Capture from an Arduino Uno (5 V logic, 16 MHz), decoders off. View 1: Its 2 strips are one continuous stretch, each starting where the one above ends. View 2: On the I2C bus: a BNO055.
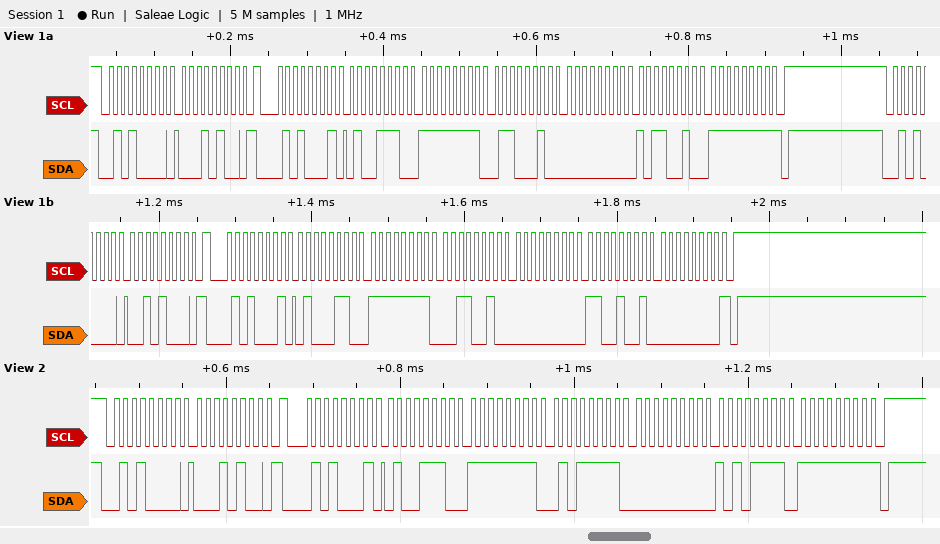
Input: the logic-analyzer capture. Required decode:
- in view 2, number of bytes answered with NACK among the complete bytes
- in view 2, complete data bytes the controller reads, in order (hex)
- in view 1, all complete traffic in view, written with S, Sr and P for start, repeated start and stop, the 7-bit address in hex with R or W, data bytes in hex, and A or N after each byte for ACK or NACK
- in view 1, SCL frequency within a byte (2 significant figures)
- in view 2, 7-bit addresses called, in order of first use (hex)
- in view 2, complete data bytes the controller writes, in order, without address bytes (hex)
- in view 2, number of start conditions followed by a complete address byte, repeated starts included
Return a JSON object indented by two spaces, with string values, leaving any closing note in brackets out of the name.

{
  "in view 2, number of bytes answered with NACK among the complete bytes": "1",
  "in view 2, complete data bytes the controller reads, in order": "4E FF 5F 00 AF FF",
  "in view 1, all complete traffic in view, written with S, Sr and P for start, repeated start and stop, the 7-bit address in hex with R or W, data bytes in hex, and A or N after each byte for ACK or NACK": "S 28W A 14 A Sr 28R A 4E A FF A 62 A 00 A B2 A FF N P S 28W A 28 A Sr 28R A 46 A FF A 32 A 00 A C9 A 00 N P",
  "in view 1, SCL frequency within a byte": "100 kHz",
  "in view 2, 7-bit addresses called, in order of first use": "0x28",
  "in view 2, complete data bytes the controller writes, in order, without address bytes": "14",
  "in view 2, number of start conditions followed by a complete address byte, repeated starts included": "2"
}
